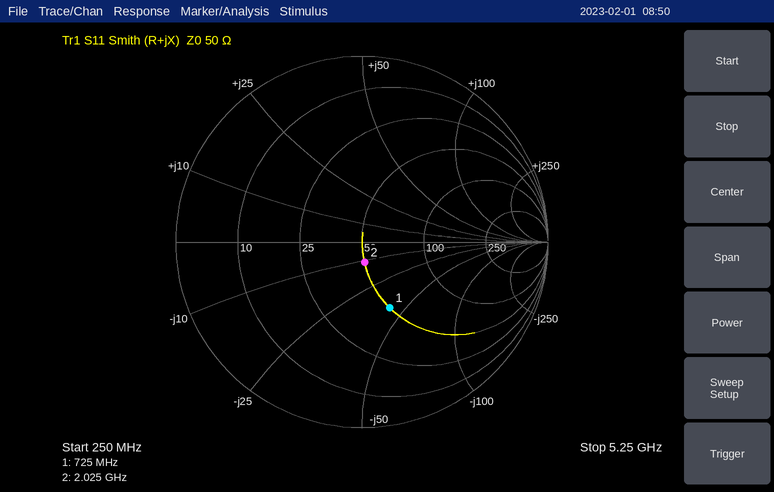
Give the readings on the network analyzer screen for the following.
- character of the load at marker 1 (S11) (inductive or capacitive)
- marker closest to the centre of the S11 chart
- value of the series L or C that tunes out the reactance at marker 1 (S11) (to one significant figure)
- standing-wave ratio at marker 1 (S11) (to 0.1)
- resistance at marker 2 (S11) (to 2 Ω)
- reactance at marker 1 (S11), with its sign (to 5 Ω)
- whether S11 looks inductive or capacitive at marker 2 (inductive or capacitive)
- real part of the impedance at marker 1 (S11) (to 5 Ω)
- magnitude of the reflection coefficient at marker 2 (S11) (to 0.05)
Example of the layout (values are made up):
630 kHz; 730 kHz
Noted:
capacitive; marker 2; 9 nH; 2.2; 50 Ω; -40 Ω; capacitive; 50 Ω; 0.10
